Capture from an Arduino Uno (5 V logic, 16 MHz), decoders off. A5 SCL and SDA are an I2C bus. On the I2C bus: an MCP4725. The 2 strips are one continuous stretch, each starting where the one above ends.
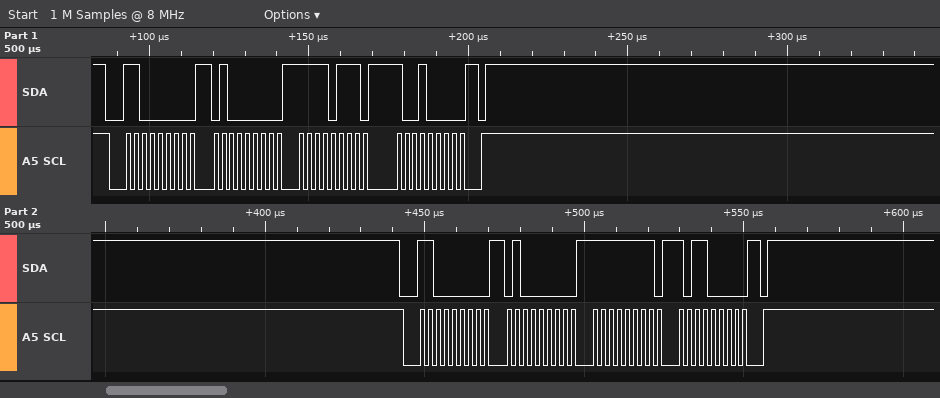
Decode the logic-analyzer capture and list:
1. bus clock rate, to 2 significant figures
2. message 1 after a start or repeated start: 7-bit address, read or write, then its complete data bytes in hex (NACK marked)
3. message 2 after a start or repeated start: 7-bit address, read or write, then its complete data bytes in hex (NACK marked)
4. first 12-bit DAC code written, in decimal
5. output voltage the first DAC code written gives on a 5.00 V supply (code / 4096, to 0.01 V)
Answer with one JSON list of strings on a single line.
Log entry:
["400 kHz", "0x60 write: 40 F7 90", "0x60 write: 40 FF B0", "3961", "4.84 V"]
